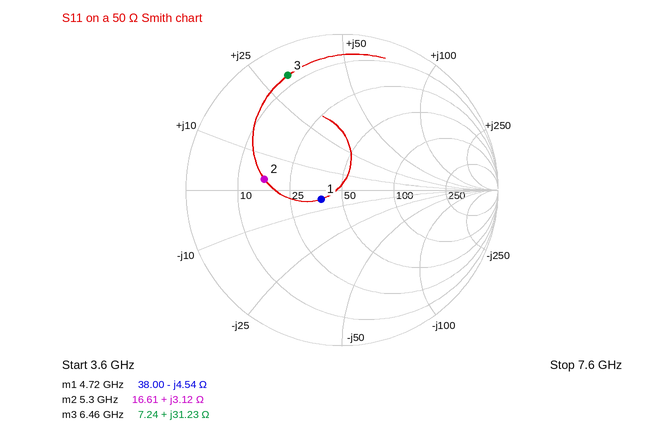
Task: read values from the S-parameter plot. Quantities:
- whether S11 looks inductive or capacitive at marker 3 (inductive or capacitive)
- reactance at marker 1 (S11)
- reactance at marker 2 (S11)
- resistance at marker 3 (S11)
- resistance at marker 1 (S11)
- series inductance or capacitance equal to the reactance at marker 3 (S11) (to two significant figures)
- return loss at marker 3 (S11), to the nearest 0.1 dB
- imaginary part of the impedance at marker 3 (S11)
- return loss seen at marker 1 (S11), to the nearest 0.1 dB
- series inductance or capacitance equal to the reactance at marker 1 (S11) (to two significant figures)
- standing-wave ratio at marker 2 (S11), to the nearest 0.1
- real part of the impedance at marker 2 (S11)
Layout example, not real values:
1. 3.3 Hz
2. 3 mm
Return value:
1. inductive
2. -4.54 Ω
3. +3.12 Ω
4. 7.24 Ω
5. 38.00 Ω
6. 770 pH
7. 1.8 dB
8. +31.23 Ω
9. 16.7 dB
10. 7.4 pF
11. 3.0
12. 16.61 Ω
